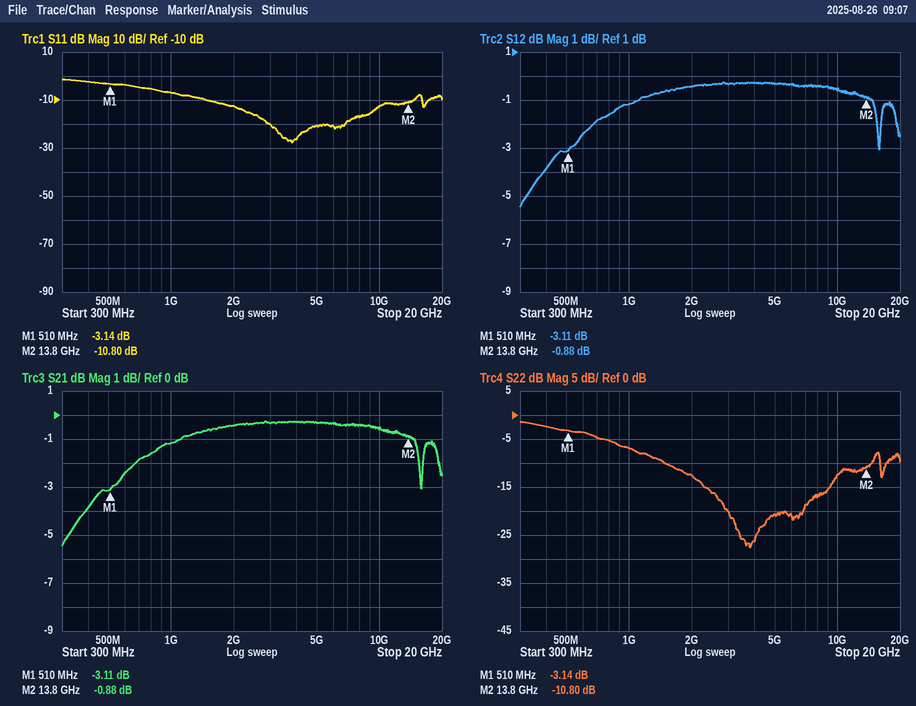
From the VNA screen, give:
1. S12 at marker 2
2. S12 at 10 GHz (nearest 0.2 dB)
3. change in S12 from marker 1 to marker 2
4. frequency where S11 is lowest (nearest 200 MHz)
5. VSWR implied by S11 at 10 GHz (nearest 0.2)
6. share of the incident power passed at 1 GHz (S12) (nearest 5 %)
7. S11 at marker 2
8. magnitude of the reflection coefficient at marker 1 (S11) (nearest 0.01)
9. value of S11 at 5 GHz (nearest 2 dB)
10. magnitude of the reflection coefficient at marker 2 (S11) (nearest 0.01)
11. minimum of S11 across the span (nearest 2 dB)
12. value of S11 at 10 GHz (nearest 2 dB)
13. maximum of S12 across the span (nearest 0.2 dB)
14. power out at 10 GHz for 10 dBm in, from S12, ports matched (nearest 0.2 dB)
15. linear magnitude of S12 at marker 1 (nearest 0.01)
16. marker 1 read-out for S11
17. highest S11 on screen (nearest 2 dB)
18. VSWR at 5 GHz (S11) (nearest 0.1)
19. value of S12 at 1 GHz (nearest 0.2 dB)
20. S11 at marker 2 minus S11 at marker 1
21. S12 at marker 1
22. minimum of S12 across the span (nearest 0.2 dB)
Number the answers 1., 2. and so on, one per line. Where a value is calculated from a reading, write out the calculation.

1. -0.88 dB
2. -0.6 dB
3. -0.88 − (-3.11) = 2.23 dB
4. 3.8 GHz
5. |Γ| = 10^(-12/20) = 0.2512; VSWR = (1 + 0.2512)/(1 − 0.2512) ≈ 1.67, so 1.6 to the nearest 0.2
6. 10^(-1.2/10) ≈ 75.9 %, so 75 % to the nearest 5 %
7. -10.80 dB
8. 10^(-3.14/20) ≈ 0.70
9. -20 dB
10. 10^(-10.8/20) ≈ 0.29
11. -28 dB
12. -12 dB
13. -0.2 dB
14. 10 dBm + (-0.6 dB) = 9.4 dBm
15. 10^(-3.11/20) ≈ 0.70
16. -3.14 dB
17. -2 dB
18. |Γ| = 10^(-20/20) = 0.1000; VSWR = (1 + 0.1000)/(1 − 0.1000) ≈ 1.2
19. -1.2 dB
20. -10.8 − (-3.14) = -7.66 dB
21. -3.11 dB
22. -5.4 dB
